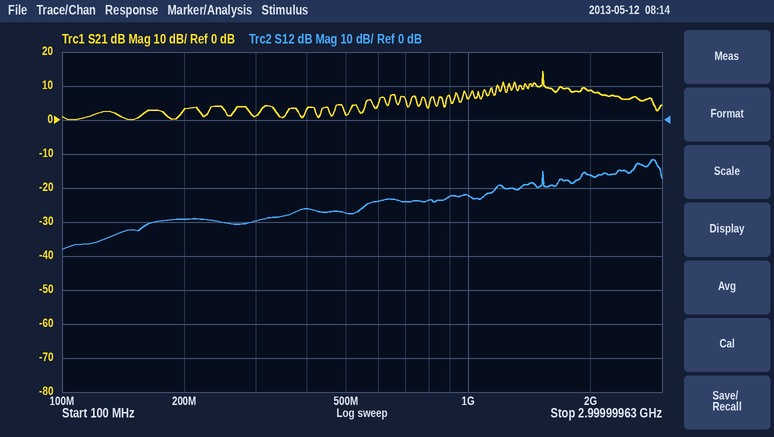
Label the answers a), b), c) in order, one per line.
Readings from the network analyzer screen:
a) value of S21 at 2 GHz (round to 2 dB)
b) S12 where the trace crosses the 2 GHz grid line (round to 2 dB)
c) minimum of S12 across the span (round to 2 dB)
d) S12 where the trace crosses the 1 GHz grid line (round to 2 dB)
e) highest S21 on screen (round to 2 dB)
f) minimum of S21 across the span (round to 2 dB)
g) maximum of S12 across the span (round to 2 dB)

a) 8 dB
b) -16 dB
c) -38 dB
d) -22 dB
e) 14 dB
f) 0 dB
g) -12 dB
